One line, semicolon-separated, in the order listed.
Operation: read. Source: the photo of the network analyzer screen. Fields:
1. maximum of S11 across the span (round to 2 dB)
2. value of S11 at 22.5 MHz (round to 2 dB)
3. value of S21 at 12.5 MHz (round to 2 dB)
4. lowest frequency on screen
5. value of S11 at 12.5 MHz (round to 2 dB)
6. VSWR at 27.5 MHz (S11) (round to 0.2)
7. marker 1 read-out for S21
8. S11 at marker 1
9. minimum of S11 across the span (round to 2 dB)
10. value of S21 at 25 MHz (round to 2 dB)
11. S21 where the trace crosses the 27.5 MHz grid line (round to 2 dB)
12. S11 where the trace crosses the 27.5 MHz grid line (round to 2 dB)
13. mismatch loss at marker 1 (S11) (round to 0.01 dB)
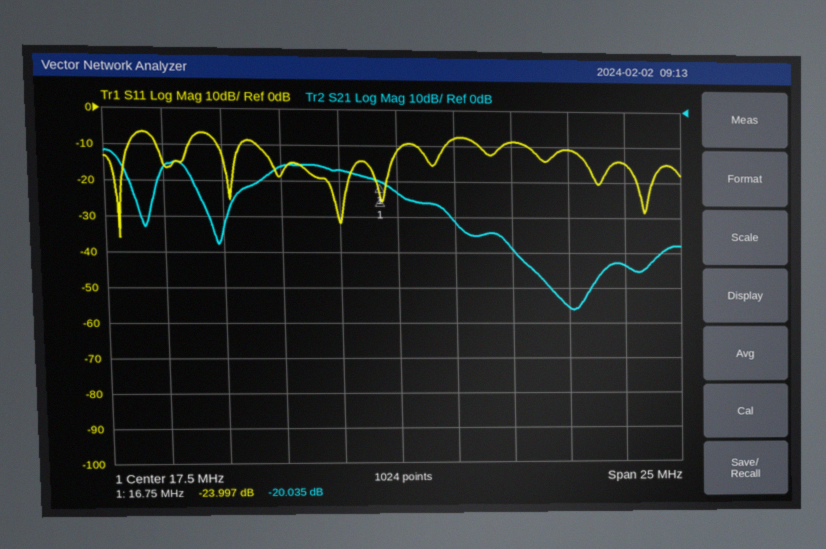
-6 dB; -8 dB; -16 dB; 5 MHz; -18 dB; 1.4; -20.035 dB; -23.997 dB; -36 dB; -56 dB; -44 dB; -14 dB; 0.02 dB
